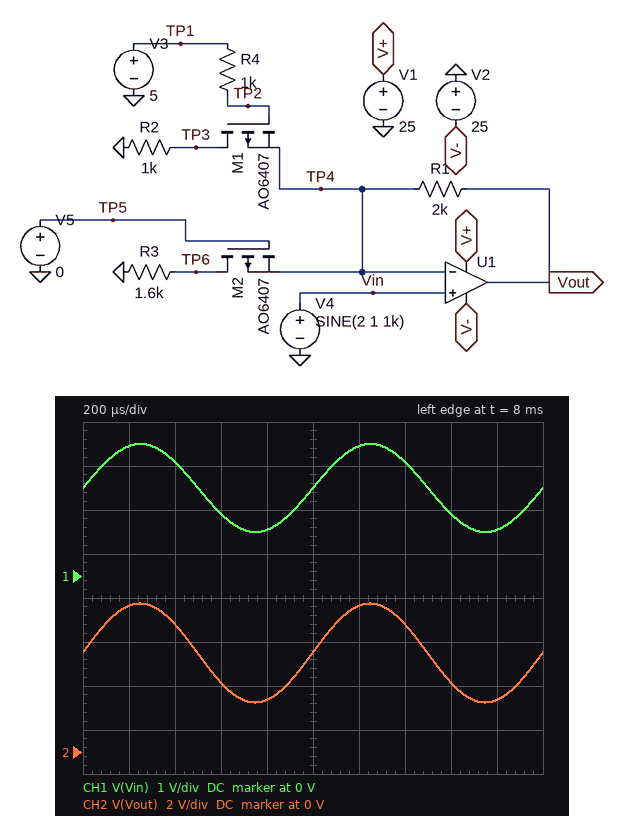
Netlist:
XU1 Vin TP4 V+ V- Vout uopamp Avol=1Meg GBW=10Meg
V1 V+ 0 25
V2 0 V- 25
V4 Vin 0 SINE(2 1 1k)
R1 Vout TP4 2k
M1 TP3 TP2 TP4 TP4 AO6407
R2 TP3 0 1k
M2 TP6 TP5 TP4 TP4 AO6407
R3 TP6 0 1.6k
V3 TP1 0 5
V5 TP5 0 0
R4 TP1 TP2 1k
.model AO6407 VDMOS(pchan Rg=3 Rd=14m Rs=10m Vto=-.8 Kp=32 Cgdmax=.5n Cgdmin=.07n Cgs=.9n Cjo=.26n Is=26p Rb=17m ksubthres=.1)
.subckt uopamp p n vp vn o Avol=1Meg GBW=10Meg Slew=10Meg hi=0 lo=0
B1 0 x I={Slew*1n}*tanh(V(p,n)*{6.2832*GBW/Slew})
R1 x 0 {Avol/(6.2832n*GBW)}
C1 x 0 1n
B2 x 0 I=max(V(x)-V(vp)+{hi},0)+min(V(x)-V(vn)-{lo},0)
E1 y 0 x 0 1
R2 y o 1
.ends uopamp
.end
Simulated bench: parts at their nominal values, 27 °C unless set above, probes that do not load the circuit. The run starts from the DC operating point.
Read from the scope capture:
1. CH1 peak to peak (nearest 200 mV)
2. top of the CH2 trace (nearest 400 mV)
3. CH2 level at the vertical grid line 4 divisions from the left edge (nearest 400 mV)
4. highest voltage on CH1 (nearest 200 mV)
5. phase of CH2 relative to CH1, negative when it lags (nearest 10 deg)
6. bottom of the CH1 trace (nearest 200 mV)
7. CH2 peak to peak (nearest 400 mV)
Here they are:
2.0 V
6.8 V
2.4 V
3.0 V
0 deg
1.0 V
4.4 V
